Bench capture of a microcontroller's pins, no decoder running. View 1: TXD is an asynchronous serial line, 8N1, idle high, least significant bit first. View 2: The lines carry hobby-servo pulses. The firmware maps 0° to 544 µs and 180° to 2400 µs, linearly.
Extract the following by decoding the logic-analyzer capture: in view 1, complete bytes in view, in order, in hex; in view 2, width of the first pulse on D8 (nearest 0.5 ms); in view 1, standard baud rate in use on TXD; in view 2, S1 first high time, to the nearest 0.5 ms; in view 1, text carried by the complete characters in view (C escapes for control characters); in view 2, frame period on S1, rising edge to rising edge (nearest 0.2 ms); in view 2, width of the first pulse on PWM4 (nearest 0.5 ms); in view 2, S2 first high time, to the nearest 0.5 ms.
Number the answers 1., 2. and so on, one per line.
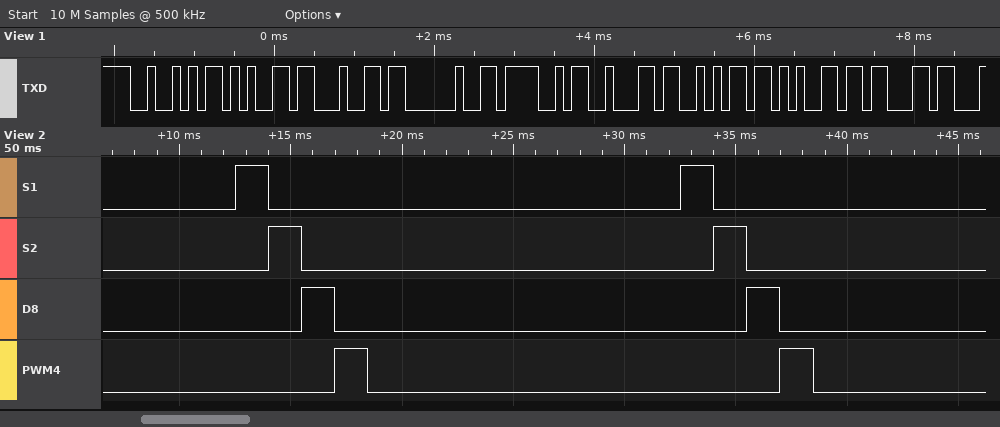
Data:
1. 52 65 64 20 4F 62 6A 65 63
2. 1.5 ms
3. 9600 baud
4. 1.5 ms
5. "Red Objec"
6. 20.0 ms
7. 1.5 ms
8. 1.5 ms
